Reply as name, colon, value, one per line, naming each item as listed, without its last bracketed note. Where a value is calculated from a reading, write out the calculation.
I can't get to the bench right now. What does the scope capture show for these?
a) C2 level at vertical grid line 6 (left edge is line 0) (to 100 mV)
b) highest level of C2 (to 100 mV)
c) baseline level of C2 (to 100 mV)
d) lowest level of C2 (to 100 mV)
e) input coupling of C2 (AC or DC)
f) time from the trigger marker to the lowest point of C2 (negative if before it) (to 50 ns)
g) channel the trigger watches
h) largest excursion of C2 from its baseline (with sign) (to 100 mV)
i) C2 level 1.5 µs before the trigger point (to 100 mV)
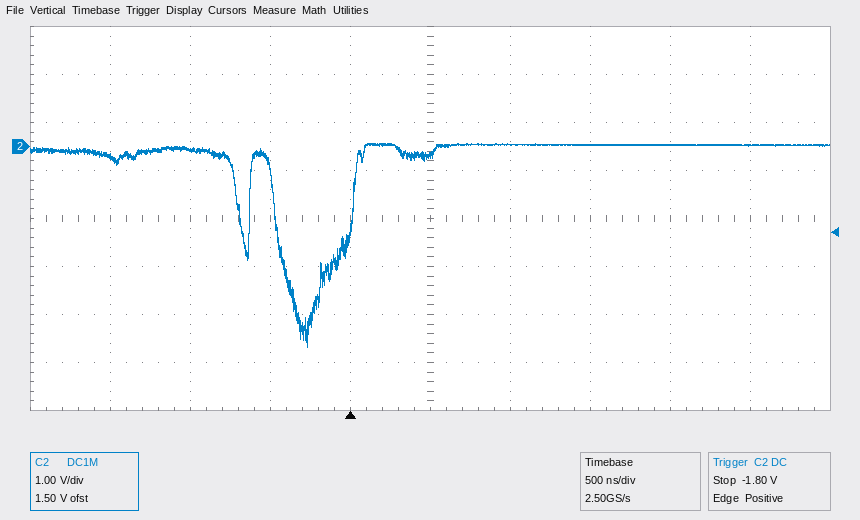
C2 level at vertical grid line 6 (left edge is line 0): 0.0 V
highest level of C2: 100 mV
baseline level of C2: 0.0 V
lowest level of C2: -4.2 V
input coupling of C2: DC
time from the trigger marker to the lowest point of C2 (negative if before it): -250 ns
channel the trigger watches: C2
largest excursion of C2 from its baseline (with sign): -4.2 V − (0.0 V) = -4.2 V
C2 level 1.5 µs before the trigger point: -200 mV
